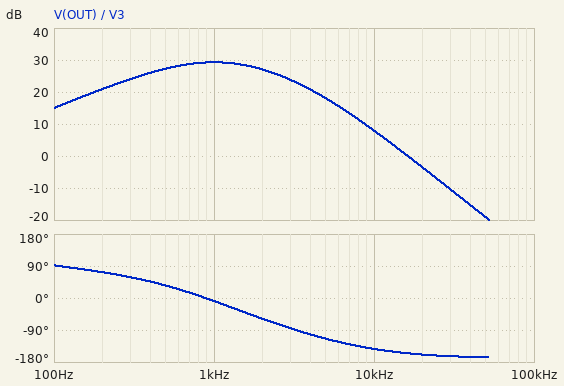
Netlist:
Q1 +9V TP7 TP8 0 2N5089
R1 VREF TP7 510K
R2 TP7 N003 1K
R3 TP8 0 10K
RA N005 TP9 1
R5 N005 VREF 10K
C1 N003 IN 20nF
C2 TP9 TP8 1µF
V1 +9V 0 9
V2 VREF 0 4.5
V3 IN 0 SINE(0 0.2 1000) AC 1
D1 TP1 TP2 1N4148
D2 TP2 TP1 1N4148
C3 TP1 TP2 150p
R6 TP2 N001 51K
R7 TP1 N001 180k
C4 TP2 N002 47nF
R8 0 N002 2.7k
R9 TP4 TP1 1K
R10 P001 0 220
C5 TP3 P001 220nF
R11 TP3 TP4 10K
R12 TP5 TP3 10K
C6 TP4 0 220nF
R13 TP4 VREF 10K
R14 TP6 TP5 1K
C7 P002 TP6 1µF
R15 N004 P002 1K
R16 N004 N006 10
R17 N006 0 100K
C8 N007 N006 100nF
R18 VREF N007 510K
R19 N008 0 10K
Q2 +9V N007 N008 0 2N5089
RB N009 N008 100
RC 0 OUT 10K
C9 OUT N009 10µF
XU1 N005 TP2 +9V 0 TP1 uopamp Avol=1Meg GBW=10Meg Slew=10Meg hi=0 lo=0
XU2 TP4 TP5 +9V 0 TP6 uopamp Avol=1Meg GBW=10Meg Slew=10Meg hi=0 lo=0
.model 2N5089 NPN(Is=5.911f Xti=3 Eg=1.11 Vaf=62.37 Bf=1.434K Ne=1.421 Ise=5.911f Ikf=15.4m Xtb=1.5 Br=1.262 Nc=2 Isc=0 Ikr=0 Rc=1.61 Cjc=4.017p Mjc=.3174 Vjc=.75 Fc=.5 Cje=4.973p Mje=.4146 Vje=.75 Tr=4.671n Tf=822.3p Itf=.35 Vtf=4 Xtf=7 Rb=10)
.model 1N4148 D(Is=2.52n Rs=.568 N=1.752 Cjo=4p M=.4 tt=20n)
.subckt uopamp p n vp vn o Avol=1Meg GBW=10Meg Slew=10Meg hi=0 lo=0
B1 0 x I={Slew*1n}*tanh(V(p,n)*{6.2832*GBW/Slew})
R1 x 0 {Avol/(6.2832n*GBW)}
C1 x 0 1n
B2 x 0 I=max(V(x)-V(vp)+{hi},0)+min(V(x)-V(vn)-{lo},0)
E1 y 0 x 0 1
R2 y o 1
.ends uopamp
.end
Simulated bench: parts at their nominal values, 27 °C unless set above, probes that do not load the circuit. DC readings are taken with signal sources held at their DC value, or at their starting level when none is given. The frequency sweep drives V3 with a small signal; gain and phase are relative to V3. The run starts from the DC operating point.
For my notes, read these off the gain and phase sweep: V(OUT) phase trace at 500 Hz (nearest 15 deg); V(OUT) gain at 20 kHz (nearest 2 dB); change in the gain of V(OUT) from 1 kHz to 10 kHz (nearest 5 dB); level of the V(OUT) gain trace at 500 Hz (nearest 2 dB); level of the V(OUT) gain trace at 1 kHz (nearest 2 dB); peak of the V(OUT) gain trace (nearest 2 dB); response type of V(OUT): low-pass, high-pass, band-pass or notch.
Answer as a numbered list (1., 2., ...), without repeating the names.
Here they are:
1. 30 deg
2. -4 dB
3. -20 dB
4. 28 dB
5. 30 dB
6. 30 dB
7. band-pass
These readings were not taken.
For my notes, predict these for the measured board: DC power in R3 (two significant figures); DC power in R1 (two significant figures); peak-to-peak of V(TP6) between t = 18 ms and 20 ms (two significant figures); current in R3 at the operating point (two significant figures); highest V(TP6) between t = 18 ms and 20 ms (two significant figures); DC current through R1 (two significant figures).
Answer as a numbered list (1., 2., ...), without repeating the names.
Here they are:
1. 1.3 mW
2. 110 nW
3. 870 mV
4. 360 µA
5. 4.9 V
6. 460 nA
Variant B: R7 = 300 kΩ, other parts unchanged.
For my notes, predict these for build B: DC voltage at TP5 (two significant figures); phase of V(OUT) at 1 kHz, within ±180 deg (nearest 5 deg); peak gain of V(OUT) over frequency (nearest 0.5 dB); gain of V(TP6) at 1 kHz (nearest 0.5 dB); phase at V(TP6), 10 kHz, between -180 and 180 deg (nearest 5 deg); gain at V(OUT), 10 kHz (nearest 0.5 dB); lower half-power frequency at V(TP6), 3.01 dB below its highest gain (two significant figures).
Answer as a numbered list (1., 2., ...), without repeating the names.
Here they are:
1. 4.5 V
2. -15 deg
3. 32.5 dB
4. 33.0 dB
5. -150 deg
6. 8.5 dB
7. 410 Hz
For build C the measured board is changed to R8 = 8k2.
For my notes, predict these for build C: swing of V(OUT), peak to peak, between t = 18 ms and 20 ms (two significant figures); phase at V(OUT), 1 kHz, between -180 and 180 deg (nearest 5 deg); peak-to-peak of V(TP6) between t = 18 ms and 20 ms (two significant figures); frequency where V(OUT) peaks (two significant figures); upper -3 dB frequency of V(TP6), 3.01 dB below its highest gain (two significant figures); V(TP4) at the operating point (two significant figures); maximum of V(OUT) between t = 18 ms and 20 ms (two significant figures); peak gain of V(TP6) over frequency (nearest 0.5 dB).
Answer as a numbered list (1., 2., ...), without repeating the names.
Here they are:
1. 790 mV
2. -35 deg
3. 820 mV
4. 590 Hz
5. 1.4 kHz
6. 4.5 V
7. 390 mV
8. 24.5 dB
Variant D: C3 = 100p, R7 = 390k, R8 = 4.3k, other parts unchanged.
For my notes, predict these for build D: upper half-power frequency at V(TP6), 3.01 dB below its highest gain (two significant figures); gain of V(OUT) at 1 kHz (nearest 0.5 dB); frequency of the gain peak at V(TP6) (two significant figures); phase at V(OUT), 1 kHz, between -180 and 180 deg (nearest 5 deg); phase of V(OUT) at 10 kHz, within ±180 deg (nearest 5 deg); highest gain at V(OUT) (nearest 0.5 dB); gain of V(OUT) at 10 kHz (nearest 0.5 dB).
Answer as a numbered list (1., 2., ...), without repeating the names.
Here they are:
1. 1.8 kHz
2. 32.5 dB
3. 790 Hz
4. -25 deg
5. -150 deg
6. 33.0 dB
7. 7.5 dB
